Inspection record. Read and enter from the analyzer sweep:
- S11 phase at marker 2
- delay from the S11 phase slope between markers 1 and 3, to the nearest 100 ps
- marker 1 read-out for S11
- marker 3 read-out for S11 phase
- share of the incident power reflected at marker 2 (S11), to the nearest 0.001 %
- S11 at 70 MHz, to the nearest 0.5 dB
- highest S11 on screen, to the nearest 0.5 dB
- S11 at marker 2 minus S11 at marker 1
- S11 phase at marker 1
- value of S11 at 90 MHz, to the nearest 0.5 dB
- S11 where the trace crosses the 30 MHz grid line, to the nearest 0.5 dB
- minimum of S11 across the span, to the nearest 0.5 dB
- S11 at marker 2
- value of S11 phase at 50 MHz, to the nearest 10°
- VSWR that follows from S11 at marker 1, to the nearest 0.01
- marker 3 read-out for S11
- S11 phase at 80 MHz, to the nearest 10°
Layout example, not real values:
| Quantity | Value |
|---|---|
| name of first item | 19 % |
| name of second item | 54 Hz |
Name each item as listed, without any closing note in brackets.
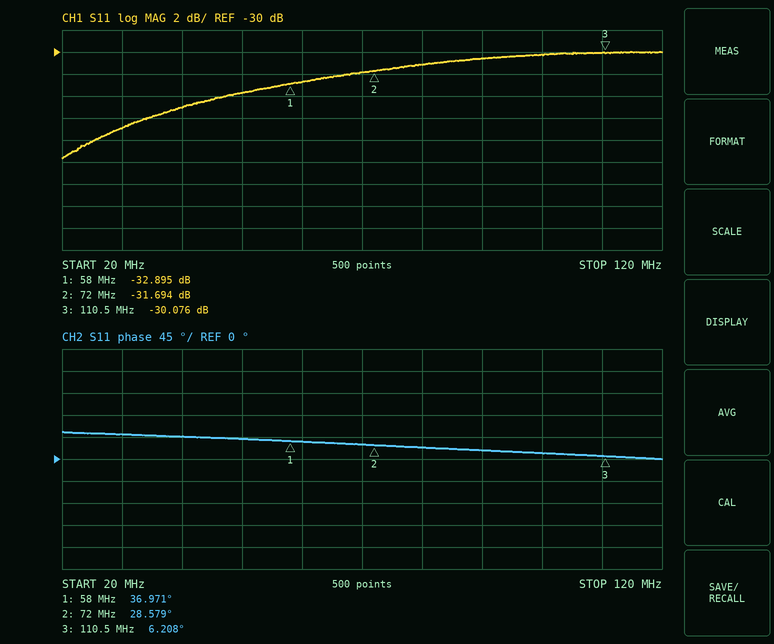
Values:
| Quantity | Value |
|---|---|
| S11 phase at marker 2 | 28.579° |
| delay from the S11 phase slope between markers 1 and 3, to the nearest 100 ps | 1.6 ns |
| marker 1 read-out for S11 | -32.895 dB |
| marker 3 read-out for S11 phase | 6.208° |
| share of the incident power reflected at marker 2 (S11), to the nearest 0.001 % | 0.068 % |
| S11 at 70 MHz, to the nearest 0.5 dB | -32.0 dB |
| highest S11 on screen, to the nearest 0.5 dB | -30.0 dB |
| S11 at marker 2 minus S11 at marker 1 | 1.201 dB |
| S11 phase at marker 1 | 36.971° |
| value of S11 at 90 MHz, to the nearest 0.5 dB | -30.5 dB |
| S11 where the trace crosses the 30 MHz grid line, to the nearest 0.5 dB | -37.0 dB |
| minimum of S11 across the span, to the nearest 0.5 dB | -39.5 dB |
| S11 at marker 2 | -31.694 dB |
| value of S11 phase at 50 MHz, to the nearest 10° | 40° |
| VSWR that follows from S11 at marker 1, to the nearest 0.01 | 1.05 |
| marker 3 read-out for S11 | -30.076 dB |
| S11 phase at 80 MHz, to the nearest 10° | 20° |
